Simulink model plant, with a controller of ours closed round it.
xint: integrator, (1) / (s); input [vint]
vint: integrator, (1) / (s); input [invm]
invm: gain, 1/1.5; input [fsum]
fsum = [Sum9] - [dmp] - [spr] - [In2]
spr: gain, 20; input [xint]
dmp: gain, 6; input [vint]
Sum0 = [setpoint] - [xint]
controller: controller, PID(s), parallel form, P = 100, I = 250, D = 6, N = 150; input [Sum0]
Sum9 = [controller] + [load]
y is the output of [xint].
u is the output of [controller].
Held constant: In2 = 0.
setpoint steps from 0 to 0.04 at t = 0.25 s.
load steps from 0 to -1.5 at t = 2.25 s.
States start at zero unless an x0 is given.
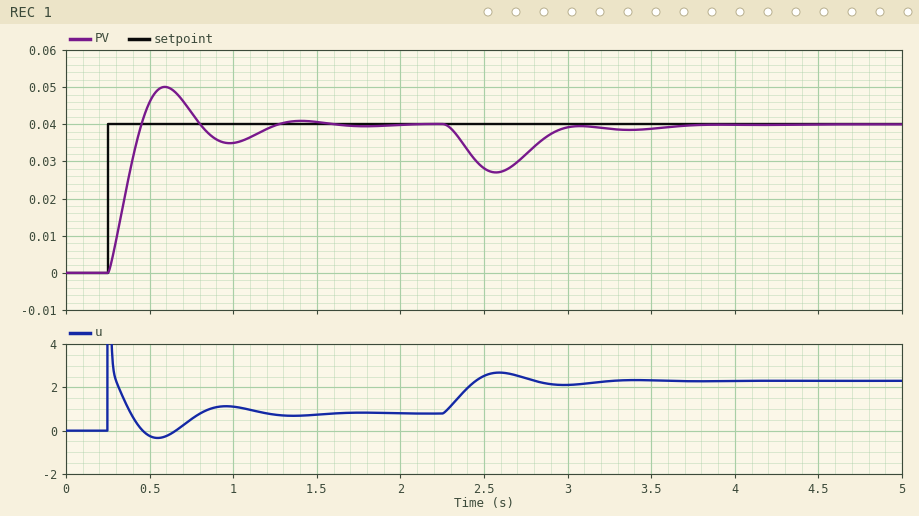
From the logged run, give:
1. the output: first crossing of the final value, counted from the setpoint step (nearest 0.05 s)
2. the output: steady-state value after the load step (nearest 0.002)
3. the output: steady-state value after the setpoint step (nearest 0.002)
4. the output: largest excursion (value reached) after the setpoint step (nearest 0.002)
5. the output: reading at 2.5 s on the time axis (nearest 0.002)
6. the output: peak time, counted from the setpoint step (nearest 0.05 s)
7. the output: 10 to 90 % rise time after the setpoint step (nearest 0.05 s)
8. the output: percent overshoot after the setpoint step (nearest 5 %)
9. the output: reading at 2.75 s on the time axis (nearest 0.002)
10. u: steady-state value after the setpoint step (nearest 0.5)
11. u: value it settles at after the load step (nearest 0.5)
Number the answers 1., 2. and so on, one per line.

1. 0.20 s
2. 0.040
3. 0.040
4. 0.050
5. 0.028
6. 0.35 s
7. 0.15 s
8. 25 %
9. 0.032
10. 1.0
11. 2.5
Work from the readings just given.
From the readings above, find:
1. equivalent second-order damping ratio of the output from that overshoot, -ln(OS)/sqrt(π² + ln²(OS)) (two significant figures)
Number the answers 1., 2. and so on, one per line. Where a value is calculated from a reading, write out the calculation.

1. ln(0.25) = -1.386; 1.386 / sqrt(9.870 + 1.922) = 0.40
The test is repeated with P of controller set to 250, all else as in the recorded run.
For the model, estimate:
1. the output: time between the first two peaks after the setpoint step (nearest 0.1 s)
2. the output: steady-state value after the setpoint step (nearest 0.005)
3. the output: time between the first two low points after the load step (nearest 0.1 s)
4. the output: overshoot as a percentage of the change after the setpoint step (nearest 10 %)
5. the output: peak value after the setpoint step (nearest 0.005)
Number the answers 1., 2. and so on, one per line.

1. 0.5 s
2. 0.040
3. 0.5 s
4. 40 %
5. 0.055
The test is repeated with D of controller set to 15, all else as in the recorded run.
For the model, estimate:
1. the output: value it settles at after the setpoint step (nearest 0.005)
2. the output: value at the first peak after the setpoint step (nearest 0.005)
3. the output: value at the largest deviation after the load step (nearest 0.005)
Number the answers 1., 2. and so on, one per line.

1. 0.040
2. 0.040
3. 0.030
